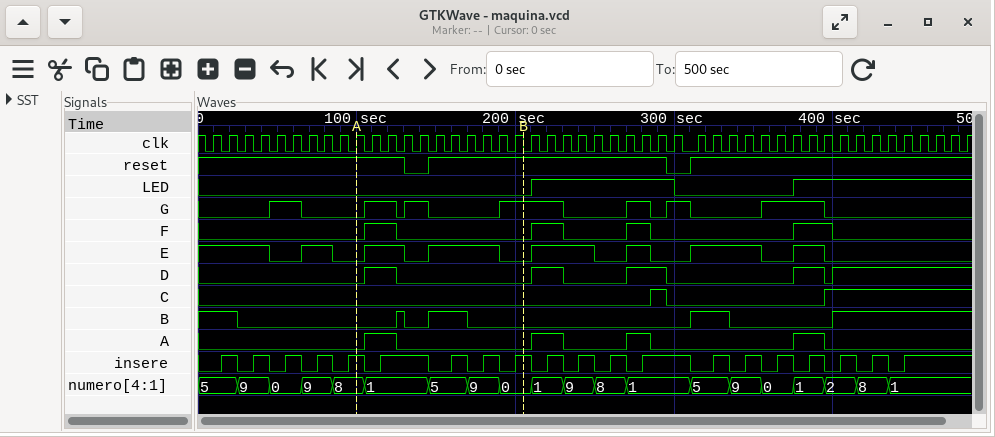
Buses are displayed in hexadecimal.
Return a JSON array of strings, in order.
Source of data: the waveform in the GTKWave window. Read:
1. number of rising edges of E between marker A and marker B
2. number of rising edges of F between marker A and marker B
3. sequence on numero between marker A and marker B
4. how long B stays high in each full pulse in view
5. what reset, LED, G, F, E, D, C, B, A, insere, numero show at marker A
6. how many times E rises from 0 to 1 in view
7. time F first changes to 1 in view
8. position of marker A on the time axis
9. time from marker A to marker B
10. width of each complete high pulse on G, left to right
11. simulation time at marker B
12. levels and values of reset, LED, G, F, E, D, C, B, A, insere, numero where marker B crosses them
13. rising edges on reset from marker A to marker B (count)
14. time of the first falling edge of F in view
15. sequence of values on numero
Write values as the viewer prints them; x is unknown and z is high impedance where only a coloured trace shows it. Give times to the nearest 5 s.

["2", "1", "8, 1, 5, 9, 0", "5 s, 25 s, 25 s", "reset=1, LED=0, G=0, F=0, E=0, D=0, C=0, B=0, A=0, insere=1, numero=8", "7", "105 s", "100 s", "105 s", "20 s, 20 s, 15 s, 40 s, 15 s, 15 s, 40 s", "205 s", "reset=1, LED=0, G=1, F=0, E=0, D=0, C=0, B=0, A=0, insere=1, numero=0", "1", "125 s", "5, 9, 0, 9, 8, 1, 5, 9, 0, 1, 9, 8, 1, 5, 9, 0, 1, 2, 8, 1"]
